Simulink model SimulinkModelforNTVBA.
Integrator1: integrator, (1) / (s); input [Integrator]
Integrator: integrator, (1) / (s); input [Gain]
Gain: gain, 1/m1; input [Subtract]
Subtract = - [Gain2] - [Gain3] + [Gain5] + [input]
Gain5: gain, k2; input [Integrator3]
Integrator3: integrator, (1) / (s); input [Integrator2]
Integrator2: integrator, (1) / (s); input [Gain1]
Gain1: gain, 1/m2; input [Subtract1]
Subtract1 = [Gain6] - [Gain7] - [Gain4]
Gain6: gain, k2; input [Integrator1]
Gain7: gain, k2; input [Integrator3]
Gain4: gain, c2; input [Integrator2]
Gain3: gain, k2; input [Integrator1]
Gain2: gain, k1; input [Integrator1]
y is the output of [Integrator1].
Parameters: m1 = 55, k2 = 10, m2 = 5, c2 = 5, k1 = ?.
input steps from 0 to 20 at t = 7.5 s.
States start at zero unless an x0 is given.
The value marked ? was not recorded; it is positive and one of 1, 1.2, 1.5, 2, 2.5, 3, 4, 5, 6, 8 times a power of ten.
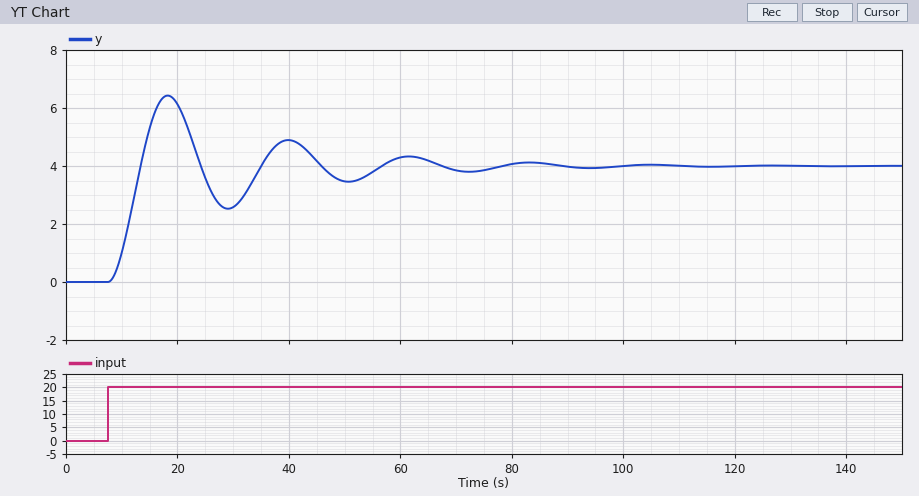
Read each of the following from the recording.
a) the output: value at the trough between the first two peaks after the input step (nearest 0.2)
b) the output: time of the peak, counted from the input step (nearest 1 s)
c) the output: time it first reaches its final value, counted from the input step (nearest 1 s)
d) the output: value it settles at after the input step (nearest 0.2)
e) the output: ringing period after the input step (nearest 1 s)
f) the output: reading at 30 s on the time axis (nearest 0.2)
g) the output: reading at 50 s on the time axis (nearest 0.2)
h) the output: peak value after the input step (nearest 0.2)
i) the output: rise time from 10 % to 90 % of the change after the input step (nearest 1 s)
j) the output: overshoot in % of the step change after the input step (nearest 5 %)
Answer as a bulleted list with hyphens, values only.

- 2.6
- 11 s
- 6 s
- 4.0
- 22 s
- 2.6
- 3.4
- 6.4
- 4 s
- 60 %
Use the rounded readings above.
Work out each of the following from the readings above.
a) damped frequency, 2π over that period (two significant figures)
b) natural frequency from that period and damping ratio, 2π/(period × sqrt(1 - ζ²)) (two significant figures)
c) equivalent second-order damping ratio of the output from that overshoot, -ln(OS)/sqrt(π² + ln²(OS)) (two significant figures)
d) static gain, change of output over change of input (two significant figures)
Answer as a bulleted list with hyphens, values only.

- 0.29 rad/s
- 0.29 rad/s
- 0.16
- 0.20
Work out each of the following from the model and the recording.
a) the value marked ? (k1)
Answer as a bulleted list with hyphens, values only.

- 5
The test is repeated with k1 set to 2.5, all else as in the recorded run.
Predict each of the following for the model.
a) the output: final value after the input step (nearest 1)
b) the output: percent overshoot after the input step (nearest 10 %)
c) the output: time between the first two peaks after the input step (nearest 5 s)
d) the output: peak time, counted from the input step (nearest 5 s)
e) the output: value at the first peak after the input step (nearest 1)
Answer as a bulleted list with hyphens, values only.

- 8
- 50 %
- 30 s
- 15 s
- 12
